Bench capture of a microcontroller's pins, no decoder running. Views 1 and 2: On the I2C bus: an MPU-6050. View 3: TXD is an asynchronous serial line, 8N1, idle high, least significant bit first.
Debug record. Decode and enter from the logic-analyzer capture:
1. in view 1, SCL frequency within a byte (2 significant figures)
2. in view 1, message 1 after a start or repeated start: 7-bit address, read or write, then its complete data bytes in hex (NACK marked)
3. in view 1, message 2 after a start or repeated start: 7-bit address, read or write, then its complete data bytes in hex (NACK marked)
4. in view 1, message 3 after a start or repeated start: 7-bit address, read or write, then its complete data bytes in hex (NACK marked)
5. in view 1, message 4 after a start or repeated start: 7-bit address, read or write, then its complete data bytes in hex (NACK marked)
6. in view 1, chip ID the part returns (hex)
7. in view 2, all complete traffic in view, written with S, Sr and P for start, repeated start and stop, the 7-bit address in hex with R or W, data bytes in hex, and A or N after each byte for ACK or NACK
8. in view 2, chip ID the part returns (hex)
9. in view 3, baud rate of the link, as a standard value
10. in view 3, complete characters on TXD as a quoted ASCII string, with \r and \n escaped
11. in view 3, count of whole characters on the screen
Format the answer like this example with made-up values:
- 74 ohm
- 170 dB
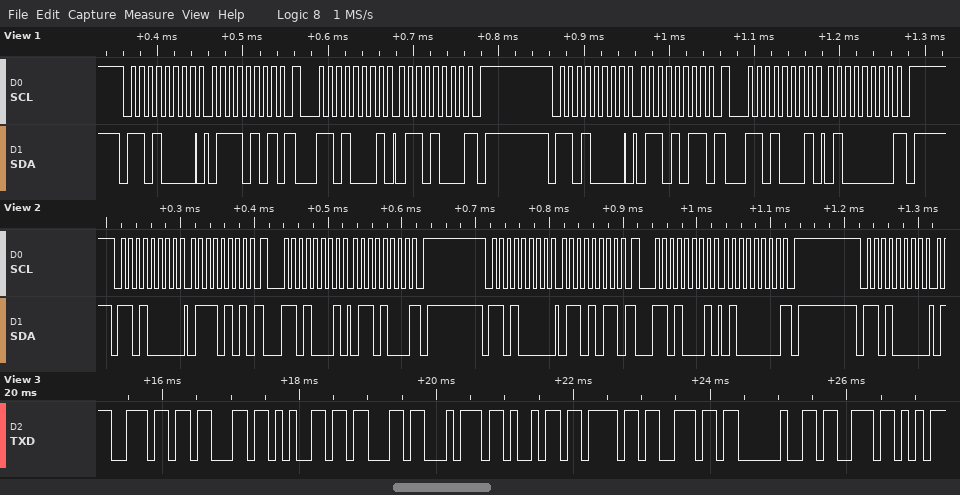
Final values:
- 100 kHz
- 0x68 write: 75
- 0x68 read: 68 NACK
- 0x68 write: 6B
- 0x68 read: 40 NACK
- 0x68
- S 68W A 75 A Sr 68R A 68 N P S 68W A 6B A Sr 68R A 40 N P S 68W A
- 0x68
- 9600 baud
- "ncection s"
- 10
